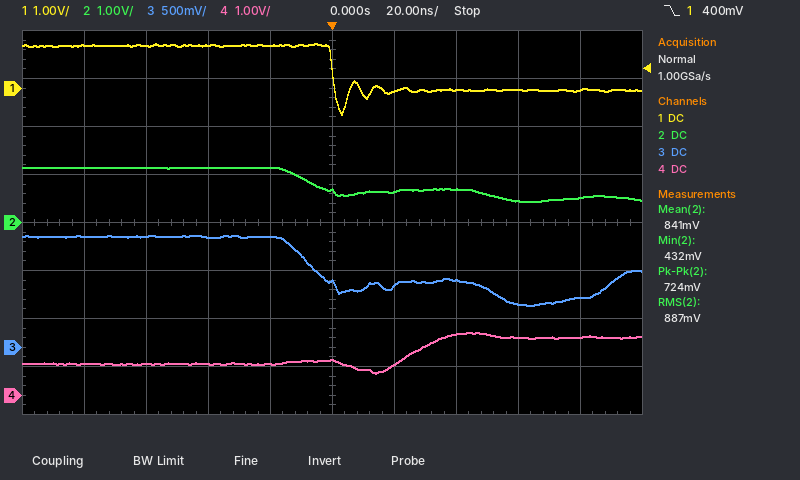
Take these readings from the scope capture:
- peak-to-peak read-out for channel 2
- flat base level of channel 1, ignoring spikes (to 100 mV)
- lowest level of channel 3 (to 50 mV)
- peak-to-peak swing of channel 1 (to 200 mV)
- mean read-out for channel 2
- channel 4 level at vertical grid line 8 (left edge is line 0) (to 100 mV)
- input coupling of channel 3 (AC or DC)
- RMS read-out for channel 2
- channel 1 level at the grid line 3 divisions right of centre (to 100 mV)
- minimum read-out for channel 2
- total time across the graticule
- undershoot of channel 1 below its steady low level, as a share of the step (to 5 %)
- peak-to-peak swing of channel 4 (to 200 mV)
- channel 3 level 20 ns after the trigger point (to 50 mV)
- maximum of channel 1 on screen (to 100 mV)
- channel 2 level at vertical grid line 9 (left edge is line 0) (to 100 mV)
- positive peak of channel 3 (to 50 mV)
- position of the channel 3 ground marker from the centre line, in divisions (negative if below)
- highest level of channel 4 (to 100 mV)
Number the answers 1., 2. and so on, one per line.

1. 724 mV
2. 0.0 V
3. 450 mV
4. 1.4 V
5. 841 mV
6. 1.2 V
7. DC
8. 887 mV
9. 0.0 V
10. 432 mV
11. 200 ns
12. 55 %
13. 800 mV
14. 650 mV
15. 900 mV
16. 500 mV
17. 1.15 V
18. -2.6 div
19. 1.3 V
